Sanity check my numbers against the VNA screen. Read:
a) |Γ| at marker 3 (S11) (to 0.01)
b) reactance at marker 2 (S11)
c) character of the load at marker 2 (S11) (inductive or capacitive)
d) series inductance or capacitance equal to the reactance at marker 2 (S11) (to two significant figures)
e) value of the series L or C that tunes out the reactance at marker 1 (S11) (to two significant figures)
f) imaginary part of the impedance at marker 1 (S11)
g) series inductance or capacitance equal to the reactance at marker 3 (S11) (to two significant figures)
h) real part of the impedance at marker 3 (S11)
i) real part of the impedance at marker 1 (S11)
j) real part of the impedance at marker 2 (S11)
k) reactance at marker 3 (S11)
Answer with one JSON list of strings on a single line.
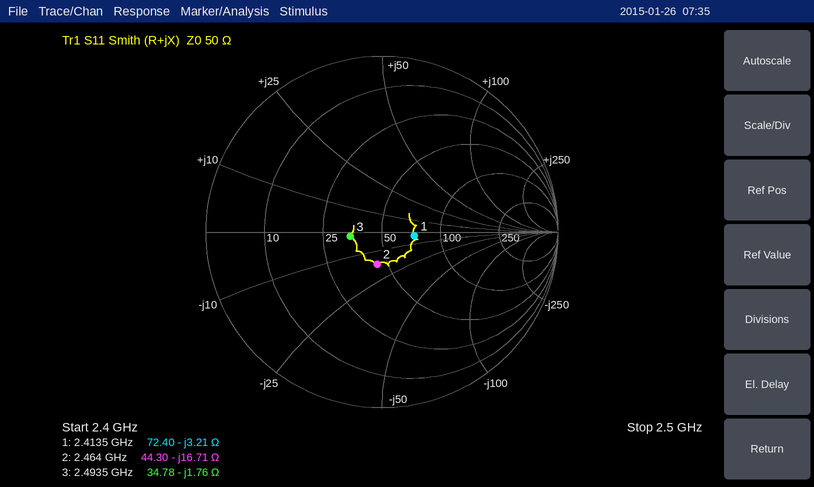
["0.18", "-16.71 Ω", "capacitive", "3.9 pF", "210 pH", "-3.21 Ω", "36 pF", "34.78 Ω", "72.40 Ω", "44.30 Ω", "-1.76 Ω"]
